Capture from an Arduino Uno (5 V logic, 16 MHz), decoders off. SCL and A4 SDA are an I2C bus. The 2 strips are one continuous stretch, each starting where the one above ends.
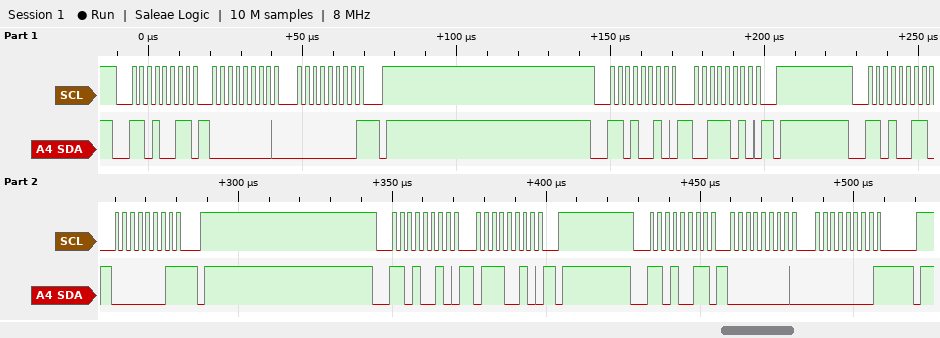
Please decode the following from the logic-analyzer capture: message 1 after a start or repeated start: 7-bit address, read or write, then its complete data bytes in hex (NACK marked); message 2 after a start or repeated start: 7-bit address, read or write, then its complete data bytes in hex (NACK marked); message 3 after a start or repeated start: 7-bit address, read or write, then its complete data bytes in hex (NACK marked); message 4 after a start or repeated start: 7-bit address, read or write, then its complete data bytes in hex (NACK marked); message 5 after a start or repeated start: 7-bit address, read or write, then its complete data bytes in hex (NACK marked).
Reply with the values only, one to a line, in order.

0x69 read: 00 00 NACK
0x69 write: 3A
0x69 read: 01 NACK
0x69 write: 72
0x69 read: 00 00 NACK
